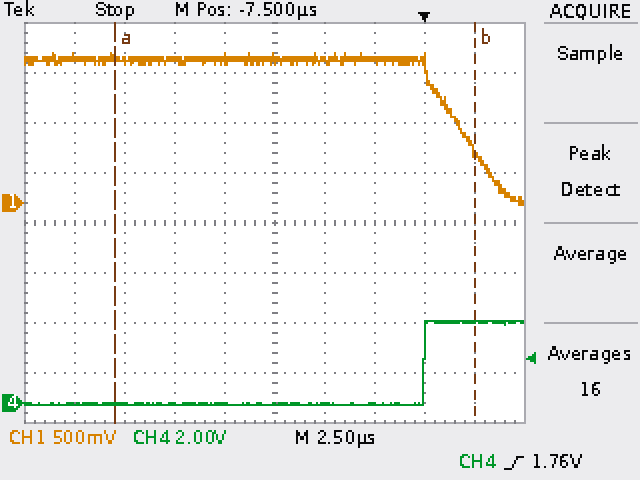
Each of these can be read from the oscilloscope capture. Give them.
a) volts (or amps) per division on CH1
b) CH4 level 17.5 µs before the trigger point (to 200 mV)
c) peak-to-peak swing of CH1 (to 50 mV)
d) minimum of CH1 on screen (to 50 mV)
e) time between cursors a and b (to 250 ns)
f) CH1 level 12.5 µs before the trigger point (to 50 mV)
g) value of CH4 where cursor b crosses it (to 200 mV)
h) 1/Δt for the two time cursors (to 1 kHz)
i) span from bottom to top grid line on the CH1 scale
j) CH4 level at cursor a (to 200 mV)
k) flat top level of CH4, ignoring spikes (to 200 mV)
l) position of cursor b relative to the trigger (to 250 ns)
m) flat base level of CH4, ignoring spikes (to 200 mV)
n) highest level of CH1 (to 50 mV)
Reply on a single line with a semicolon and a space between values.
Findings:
500 mV; 0.0 V; 1.50 V; 0 mV; 18.00 µs; 1.45 V; 3.2 V; 56 kHz; 4 V; 0.0 V; 3.2 V; +2.50 µs; 0.0 V; 1.50 V
